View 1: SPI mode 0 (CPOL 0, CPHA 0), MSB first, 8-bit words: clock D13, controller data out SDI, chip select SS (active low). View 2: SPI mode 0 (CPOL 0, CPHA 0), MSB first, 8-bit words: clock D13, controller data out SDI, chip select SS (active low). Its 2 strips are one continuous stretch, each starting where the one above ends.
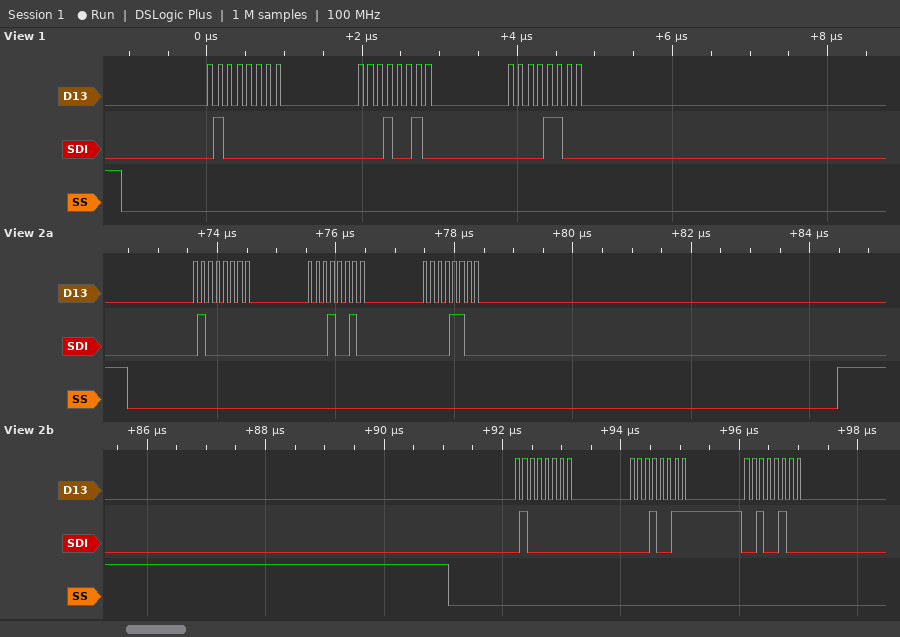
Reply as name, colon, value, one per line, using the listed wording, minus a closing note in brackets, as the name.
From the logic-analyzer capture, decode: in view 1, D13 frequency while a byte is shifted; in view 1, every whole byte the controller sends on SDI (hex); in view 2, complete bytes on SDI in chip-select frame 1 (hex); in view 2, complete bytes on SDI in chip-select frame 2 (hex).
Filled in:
in view 1, D13 frequency while a byte is shifted: 8 MHz
in view 1, every whole byte the controller sends on SDI: 40 12 0C
in view 2, complete bytes on SDI in chip-select frame 1: 40 12 0C
in view 2, complete bytes on SDI in chip-select frame 2: 40 13 24
